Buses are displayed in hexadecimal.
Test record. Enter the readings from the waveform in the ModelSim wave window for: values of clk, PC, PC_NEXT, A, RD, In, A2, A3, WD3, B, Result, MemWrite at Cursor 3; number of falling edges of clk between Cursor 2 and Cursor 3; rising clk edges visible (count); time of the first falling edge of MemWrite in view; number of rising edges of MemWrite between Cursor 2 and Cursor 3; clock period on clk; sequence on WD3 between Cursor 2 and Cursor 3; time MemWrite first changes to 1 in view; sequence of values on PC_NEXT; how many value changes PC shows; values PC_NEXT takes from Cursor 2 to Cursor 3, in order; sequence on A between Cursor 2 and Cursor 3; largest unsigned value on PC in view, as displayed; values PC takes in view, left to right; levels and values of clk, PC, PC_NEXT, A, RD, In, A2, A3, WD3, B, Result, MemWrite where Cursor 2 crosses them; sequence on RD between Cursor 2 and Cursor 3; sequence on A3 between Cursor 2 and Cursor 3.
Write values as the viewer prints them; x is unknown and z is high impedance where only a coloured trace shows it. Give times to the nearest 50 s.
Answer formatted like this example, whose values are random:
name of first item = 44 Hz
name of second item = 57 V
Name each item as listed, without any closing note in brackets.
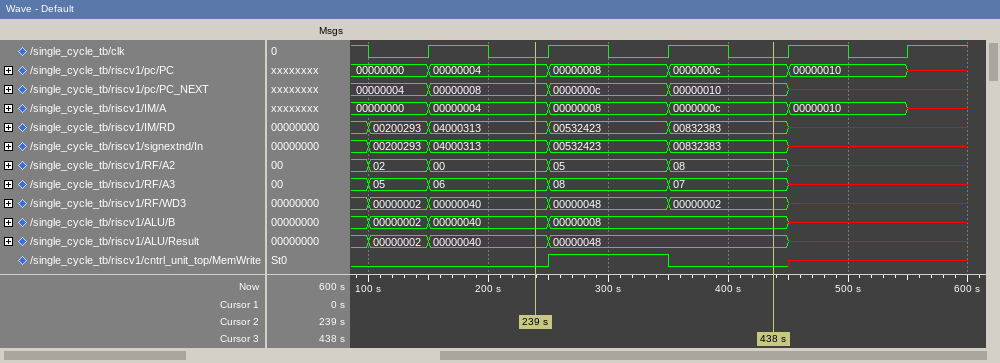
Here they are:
values of clk, PC, PC_NEXT, A, RD, In, A2, A3, WD3, B, Result, MemWrite at Cursor 3 = clk=0, PC=0000000c, PC_NEXT=00000010, A=0000000c, RD=00832383, In=00832383, A2=08, A3=07, WD3=00000002, B=00000008, Result=00000048, MemWrite=0
number of falling edges of clk between Cursor 2 and Cursor 3 = 2
rising clk edges visible = 5
time of the first falling edge of MemWrite in view = 350 s
number of rising edges of MemWrite between Cursor 2 and Cursor 3 = 1
clock period on clk = 100 s
sequence on WD3 between Cursor 2 and Cursor 3 = 00000040, 00000048, 00000002
time MemWrite first changes to 1 in view = 250 s
sequence of values on PC_NEXT = 00000004, 00000008, 0000000c, 00000010, x
how many value changes PC shows = 5
values PC_NEXT takes from Cursor 2 to Cursor 3, in order = 00000008, 0000000c, 00000010
sequence on A between Cursor 2 and Cursor 3 = 00000004, 00000008, 0000000c
largest unsigned value on PC in view, as displayed = 00000010
values PC takes in view, left to right = 00000000, 00000004, 00000008, 0000000c, 00000010, x
levels and values of clk, PC, PC_NEXT, A, RD, In, A2, A3, WD3, B, Result, MemWrite where Cursor 2 crosses them = clk=0, PC=00000004, PC_NEXT=00000008, A=00000004, RD=04000313, In=04000313, A2=00, A3=06, WD3=00000040, B=00000040, Result=00000040, MemWrite=0
sequence on RD between Cursor 2 and Cursor 3 = 04000313, 00532423, 00832383
sequence on A3 between Cursor 2 and Cursor 3 = 06, 08, 07
